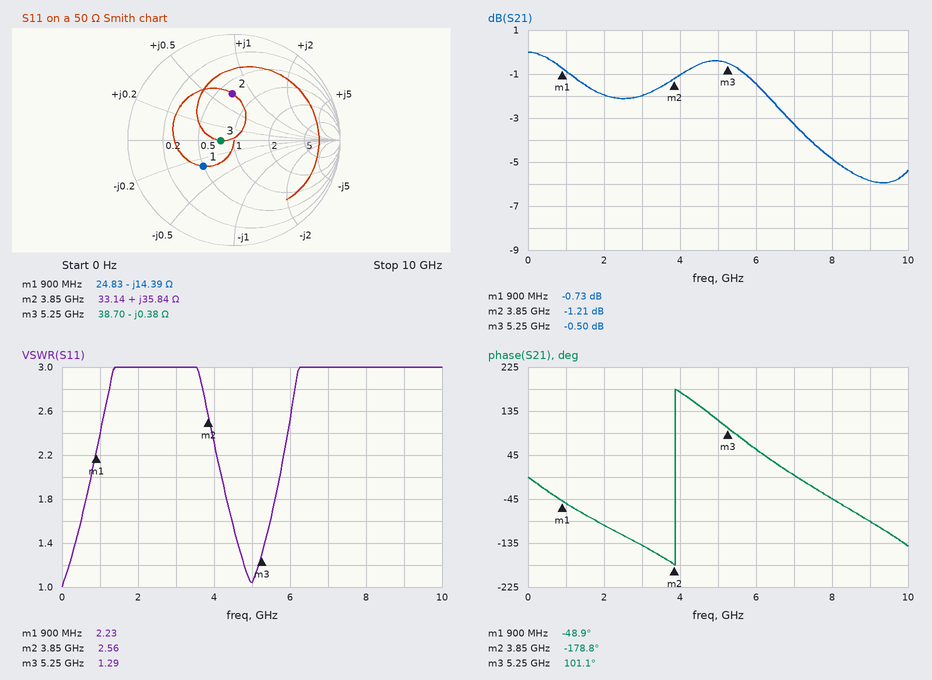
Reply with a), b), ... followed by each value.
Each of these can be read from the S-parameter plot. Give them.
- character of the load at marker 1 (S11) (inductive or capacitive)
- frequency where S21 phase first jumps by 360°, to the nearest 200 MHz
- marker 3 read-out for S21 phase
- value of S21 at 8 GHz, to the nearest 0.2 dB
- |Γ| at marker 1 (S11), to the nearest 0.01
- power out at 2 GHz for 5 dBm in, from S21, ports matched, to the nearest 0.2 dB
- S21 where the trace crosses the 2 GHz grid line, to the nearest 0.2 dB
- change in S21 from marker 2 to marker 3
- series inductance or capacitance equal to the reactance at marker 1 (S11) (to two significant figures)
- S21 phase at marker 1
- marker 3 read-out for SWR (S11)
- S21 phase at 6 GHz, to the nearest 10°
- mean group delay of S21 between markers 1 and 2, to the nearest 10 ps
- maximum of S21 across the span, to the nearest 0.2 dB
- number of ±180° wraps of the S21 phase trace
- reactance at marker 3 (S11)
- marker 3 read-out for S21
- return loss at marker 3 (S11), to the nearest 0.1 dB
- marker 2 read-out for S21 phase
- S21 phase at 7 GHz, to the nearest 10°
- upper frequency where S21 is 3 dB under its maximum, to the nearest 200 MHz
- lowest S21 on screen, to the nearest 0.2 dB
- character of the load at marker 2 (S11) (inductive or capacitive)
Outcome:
a) capacitive
b) 3.8 GHz
c) 101.1°
d) -4.8 dB
e) 0.38
f) 3.0 dBm
g) -2.0 dB
h) 0.71 dB
i) 12 pF
j) -48.9°
k) 1.29
l) 60°
m) 120 ps
n) 0.0 dB
o) 1
p) -0.38 Ω
q) -0.50 dB
r) 17.9 dB
s) -178.8°
t) 0°
u) 6.8 GHz
v) -6.0 dB
w) inductive
